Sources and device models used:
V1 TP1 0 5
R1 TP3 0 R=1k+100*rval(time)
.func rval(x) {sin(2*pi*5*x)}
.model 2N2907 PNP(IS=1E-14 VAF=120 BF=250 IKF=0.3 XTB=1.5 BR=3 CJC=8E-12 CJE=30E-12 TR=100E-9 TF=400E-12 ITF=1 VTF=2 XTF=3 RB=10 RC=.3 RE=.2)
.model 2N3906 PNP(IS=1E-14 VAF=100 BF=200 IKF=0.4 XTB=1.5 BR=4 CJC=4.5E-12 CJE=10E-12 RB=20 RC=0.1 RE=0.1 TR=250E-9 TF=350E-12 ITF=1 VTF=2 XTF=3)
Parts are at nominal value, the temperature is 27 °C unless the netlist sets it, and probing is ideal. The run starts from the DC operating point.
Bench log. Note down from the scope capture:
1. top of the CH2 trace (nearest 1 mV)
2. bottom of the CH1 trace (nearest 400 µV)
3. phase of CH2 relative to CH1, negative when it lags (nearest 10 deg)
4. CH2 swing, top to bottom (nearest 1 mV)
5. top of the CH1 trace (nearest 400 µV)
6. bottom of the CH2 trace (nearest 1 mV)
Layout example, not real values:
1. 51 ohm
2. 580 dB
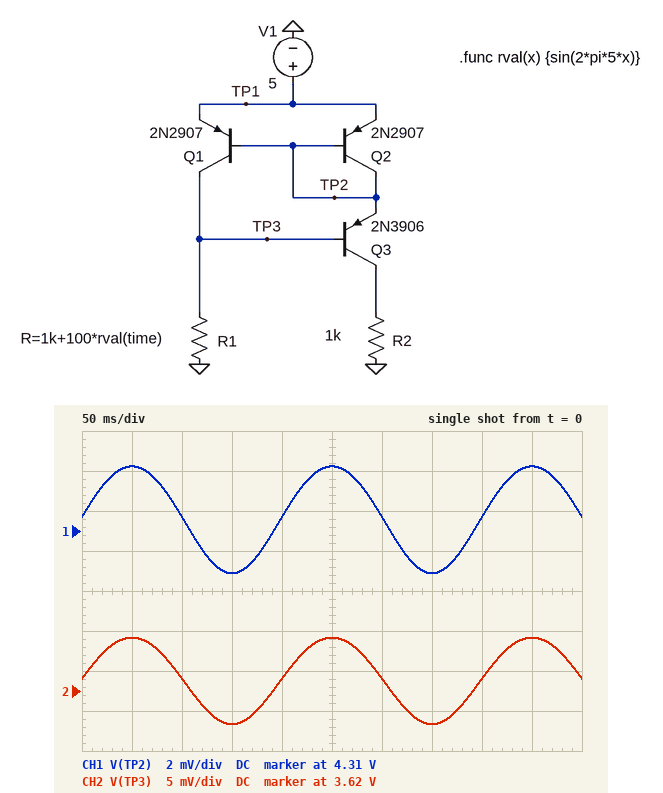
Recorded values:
1. 3.627 V
2. 4.3080 V
3. 0 deg
4. 11 mV
5. 4.3132 V
6. 3.616 V
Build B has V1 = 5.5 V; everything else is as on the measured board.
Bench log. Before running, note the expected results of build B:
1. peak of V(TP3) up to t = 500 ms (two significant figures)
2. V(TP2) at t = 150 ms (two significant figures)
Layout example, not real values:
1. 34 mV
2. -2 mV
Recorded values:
1. 4.1 V
2. 4.8 V
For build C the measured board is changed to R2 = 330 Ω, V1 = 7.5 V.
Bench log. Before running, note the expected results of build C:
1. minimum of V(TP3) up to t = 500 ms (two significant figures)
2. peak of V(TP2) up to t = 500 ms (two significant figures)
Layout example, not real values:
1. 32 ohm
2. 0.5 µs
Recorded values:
1. 6.1 V
2. 6.8 V
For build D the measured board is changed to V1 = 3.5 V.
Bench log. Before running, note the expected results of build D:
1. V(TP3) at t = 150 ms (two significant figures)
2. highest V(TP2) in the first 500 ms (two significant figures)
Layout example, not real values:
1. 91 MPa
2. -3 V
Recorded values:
1. 2.1 V
2. 2.8 V
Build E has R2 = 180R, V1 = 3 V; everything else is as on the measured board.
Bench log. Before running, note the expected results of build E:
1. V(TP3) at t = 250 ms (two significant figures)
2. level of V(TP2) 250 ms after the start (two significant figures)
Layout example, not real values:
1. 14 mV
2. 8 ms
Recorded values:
1. 1.7 V
2. 2.3 V
